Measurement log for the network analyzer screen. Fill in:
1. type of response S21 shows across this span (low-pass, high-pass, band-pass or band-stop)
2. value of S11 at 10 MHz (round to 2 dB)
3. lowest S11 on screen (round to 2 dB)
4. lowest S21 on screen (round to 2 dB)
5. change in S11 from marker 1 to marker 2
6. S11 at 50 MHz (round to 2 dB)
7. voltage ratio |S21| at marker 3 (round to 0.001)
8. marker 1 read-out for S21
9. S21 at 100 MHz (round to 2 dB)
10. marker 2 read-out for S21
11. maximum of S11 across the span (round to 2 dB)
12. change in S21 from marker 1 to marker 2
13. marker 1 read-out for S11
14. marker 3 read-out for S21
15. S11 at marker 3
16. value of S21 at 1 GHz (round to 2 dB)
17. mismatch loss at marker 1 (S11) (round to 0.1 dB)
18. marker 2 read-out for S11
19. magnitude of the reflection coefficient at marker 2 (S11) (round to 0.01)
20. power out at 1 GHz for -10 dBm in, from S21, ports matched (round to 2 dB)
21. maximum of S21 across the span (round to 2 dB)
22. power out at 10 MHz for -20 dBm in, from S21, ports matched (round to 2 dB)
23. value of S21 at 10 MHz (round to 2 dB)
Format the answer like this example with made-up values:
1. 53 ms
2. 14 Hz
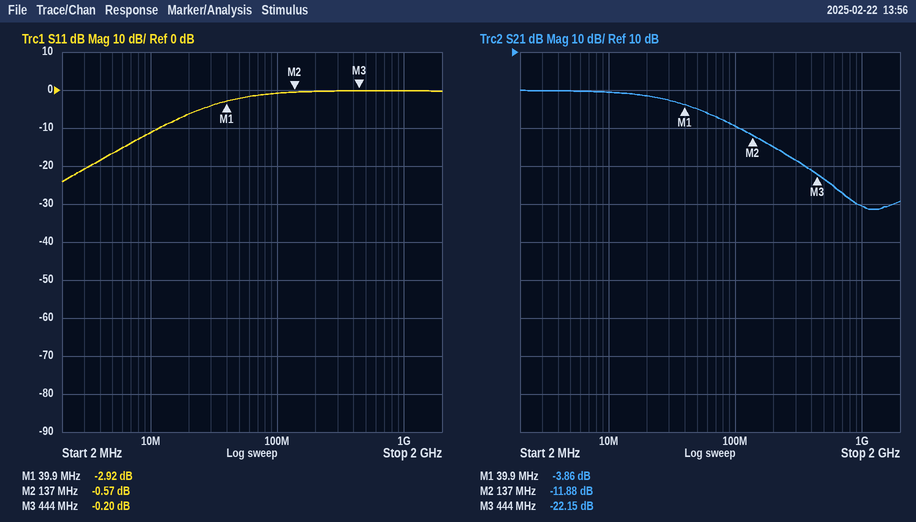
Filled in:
1. low-pass
2. -12 dB
3. -24 dB
4. -32 dB
5. 2.35 dB
6. -2 dB
7. 0.078
8. -3.86 dB
9. -10 dB
10. -11.88 dB
11. 0 dB
12. -8.02 dB
13. -2.92 dB
14. -22.15 dB
15. -0.20 dB
16. -30 dB
17. 3.1 dB
18. -0.57 dB
19. 0.94
20. -40 dBm
21. 0 dB
22. -20 dBm
23. 0 dB
